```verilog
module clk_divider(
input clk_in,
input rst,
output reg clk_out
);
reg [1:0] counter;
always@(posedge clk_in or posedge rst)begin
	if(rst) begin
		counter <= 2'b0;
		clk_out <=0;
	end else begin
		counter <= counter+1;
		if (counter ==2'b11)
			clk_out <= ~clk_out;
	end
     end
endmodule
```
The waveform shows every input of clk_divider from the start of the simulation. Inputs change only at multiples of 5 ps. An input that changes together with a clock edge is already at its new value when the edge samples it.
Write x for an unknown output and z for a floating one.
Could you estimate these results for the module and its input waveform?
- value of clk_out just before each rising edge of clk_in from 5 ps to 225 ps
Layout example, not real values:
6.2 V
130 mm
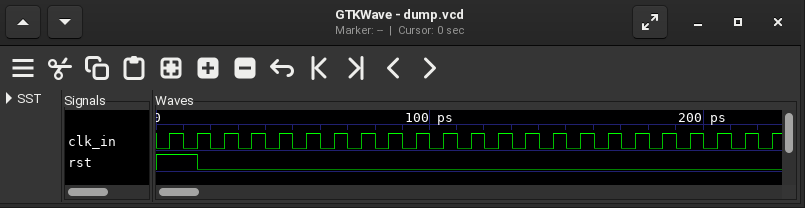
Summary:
0 0 0 0 0 1 1 1 1 0 0 0 0 1 1 1 1 0 0 0 0 1 1
